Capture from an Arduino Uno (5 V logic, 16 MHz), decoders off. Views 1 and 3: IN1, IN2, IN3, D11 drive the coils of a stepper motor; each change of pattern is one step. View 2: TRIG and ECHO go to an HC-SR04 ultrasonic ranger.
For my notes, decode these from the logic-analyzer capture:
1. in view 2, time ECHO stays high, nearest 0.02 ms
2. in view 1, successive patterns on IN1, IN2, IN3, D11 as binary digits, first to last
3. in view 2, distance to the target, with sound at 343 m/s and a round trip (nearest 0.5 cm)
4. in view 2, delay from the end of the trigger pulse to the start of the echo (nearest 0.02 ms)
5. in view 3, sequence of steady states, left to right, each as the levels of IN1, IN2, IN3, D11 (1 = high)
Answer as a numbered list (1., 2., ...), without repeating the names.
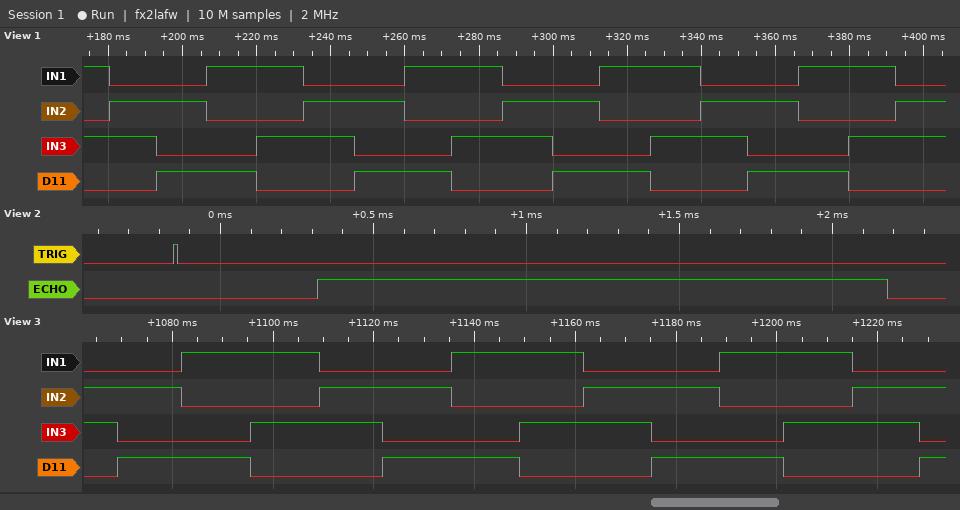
1. 1.86 ms
2. 1010 0110 0101 1001 1010 0110 0101 1001 1010 0110 0101 1001 1010 0110 0101 1001 1010 0110
3. 32 cm
4. 0.46 ms
5. 0110 0101 1001 1010 0110 0101 1001 1010 0110 0101 1001 1010 0110 0101
